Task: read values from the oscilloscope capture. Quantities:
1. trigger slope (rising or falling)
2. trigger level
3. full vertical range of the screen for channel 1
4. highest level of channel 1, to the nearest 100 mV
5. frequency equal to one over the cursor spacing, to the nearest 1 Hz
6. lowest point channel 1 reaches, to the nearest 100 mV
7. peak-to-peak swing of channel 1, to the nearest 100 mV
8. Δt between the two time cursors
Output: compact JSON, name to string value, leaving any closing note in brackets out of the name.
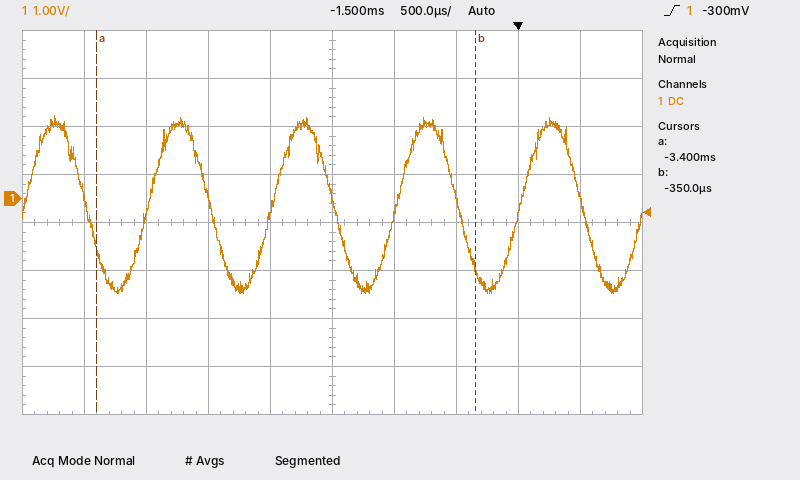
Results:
{"trigger slope": "rising", "trigger level": "-300 mV", "full vertical range of the screen for channel 1": "8 V", "highest level of channel 1, to the nearest 100 mV": "1.7 V", "frequency equal to one over the cursor spacing, to the nearest 1 Hz": "328 Hz", "lowest point channel 1 reaches, to the nearest 100 mV": "-2.0 V", "peak-to-peak swing of channel 1, to the nearest 100 mV": "3.7 V", "Δt between the two time cursors": "3.05 ms"}
